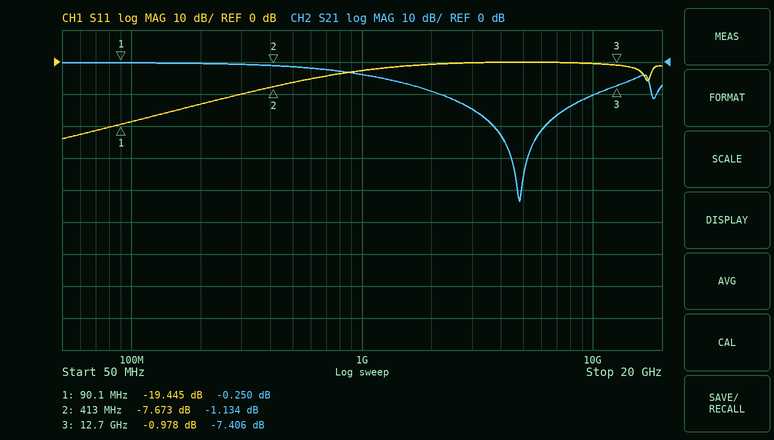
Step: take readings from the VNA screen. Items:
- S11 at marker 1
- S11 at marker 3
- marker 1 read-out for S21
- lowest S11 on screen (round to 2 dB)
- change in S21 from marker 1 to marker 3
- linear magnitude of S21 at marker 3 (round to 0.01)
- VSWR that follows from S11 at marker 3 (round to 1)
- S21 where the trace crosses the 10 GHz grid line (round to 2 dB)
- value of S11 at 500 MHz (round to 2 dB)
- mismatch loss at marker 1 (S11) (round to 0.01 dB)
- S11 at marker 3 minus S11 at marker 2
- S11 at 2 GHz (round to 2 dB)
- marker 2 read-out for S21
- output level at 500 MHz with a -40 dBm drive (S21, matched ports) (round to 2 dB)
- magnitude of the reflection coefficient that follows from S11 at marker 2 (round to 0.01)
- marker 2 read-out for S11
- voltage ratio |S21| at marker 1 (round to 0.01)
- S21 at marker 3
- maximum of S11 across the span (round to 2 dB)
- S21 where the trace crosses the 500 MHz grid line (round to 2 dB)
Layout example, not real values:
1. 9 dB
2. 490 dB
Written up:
1. -19.445 dB
2. -0.978 dB
3. -0.250 dB
4. -24 dB
5. -7.156 dB
6. 0.43
7. 18
8. -10 dB
9. -6 dB
10. 0.05 dB
11. 6.695 dB
12. 0 dB
13. -1.134 dB
14. -42 dBm
15. 0.41
16. -7.673 dB
17. 0.97
18. -7.406 dB
19. 0 dB
20. -2 dB
